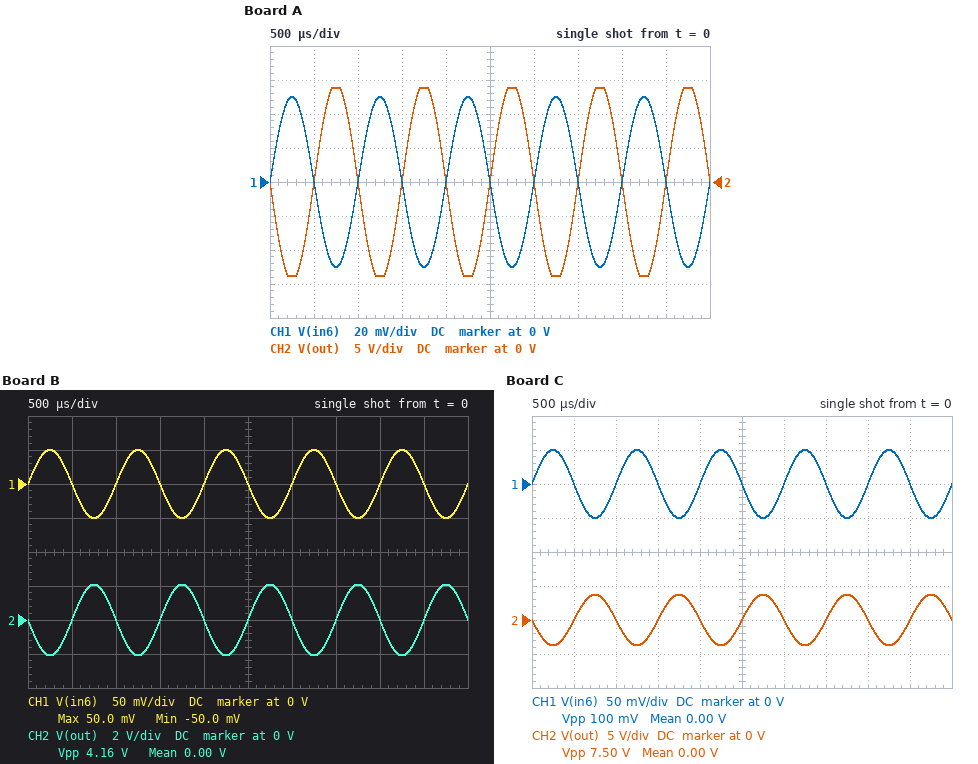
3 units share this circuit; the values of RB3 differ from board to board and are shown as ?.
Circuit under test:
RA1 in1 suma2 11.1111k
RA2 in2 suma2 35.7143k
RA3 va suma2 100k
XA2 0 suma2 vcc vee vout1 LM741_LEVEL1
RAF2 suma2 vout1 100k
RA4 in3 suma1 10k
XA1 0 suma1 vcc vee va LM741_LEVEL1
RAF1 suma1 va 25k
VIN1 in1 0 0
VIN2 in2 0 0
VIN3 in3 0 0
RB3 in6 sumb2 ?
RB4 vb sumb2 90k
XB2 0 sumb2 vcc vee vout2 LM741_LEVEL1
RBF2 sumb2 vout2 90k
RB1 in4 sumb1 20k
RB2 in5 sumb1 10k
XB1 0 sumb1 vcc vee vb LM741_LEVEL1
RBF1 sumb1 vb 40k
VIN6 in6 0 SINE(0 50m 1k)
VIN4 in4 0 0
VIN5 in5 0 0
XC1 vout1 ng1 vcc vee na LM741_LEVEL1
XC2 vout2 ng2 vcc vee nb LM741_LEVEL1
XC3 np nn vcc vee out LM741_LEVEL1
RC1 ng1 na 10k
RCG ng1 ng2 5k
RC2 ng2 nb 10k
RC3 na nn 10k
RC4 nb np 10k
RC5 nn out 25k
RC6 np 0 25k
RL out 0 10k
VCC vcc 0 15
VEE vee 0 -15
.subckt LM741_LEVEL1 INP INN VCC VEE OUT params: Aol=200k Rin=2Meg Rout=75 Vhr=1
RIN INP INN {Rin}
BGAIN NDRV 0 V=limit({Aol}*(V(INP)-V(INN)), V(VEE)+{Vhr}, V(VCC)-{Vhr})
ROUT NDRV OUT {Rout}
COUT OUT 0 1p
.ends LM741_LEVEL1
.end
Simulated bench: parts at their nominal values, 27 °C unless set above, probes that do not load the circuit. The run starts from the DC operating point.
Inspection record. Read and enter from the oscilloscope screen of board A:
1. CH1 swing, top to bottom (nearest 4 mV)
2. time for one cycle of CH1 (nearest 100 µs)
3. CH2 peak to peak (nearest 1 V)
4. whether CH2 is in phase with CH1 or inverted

100 mV
1.0 ms
28 V
inverted
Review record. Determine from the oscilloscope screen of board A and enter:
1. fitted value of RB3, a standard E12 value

3.9 kΩ
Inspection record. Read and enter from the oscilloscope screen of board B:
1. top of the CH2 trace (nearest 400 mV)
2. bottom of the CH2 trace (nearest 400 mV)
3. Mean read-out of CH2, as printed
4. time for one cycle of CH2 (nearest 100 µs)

2.0 V
-2.0 V
0.00 V
1.0 ms
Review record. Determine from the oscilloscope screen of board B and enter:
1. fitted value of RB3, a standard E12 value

27 kΩ
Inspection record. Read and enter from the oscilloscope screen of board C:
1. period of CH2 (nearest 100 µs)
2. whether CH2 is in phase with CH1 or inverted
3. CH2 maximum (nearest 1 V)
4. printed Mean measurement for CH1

1.0 ms
inverted
4 V
0.00 V
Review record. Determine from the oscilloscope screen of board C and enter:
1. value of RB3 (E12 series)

15 kΩ
